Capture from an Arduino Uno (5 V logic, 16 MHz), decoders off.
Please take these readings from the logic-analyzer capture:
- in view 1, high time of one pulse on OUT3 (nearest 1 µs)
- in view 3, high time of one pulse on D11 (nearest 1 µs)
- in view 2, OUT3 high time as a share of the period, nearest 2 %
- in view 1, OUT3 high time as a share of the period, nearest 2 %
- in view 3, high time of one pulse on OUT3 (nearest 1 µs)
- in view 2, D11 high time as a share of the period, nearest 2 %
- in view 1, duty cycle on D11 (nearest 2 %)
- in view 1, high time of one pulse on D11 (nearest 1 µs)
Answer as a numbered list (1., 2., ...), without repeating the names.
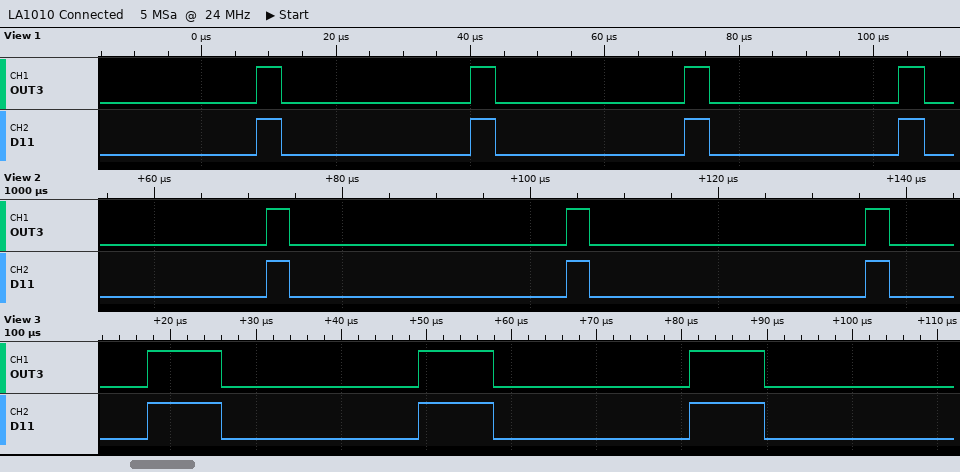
1. 4 µs
2. 9 µs
3. 8 %
4. 12 %
5. 9 µs
6. 8 %
7. 12 %
8. 4 µs
